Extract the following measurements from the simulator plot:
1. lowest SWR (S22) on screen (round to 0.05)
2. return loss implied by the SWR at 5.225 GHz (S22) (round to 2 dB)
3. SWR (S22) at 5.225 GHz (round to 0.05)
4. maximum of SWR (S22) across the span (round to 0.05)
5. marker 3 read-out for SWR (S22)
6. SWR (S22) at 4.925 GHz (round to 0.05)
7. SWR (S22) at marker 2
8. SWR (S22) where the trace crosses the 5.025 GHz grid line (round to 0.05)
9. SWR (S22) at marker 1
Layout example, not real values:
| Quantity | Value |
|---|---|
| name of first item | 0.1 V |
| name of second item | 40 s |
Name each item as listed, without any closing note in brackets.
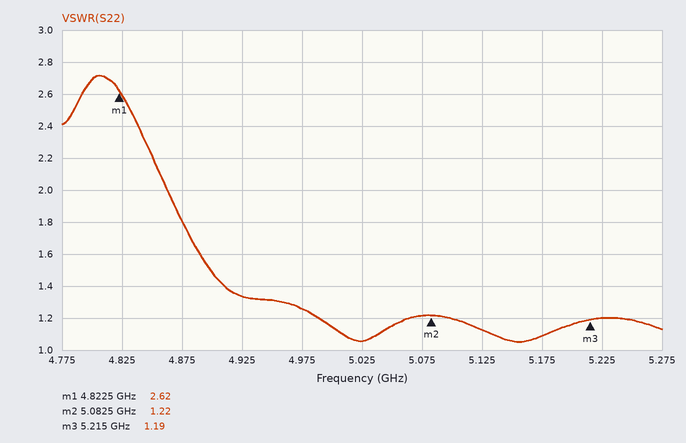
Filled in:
| Quantity | Value |
|---|---|
| lowest SWR (S22) on screen | 1.05 |
| return loss implied by the SWR at 5.225 GHz (S22) | 20 dB |
| SWR (S22) at 5.225 GHz | 1.20 |
| maximum of SWR (S22) across the span | 2.70 |
| marker 3 read-out for SWR | 1.19 |
| SWR (S22) at 4.925 GHz | 1.35 |
| SWR (S22) at marker 2 | 1.22 |
| SWR (S22) where the trace crosses the 5.025 GHz grid line | 1.05 |
| SWR (S22) at marker 1 | 2.62 |
